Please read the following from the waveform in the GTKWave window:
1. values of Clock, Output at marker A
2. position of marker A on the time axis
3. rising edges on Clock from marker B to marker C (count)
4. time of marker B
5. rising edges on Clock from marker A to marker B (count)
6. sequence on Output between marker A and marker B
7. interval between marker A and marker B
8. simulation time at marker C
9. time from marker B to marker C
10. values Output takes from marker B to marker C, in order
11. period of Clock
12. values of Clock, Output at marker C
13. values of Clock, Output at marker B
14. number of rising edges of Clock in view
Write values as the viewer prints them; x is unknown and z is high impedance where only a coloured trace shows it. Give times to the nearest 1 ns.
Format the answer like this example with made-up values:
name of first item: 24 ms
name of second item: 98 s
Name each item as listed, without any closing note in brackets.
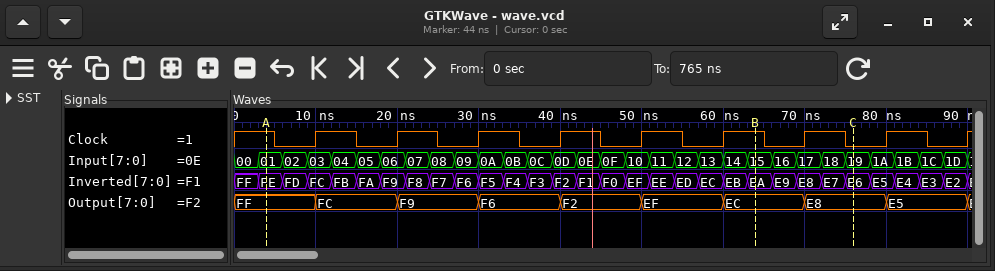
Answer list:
values of Clock, Output at marker A: Clock=1, Output=FF
position of marker A on the time axis: 4 ns
rising edges on Clock from marker B to marker C: 1
time of marker B: 64 ns
rising edges on Clock from marker A to marker B: 6
sequence on Output between marker A and marker B: FF, FC, F9, F6, F2, EF, EC
interval between marker A and marker B: 60 ns
simulation time at marker C: 76 ns
time from marker B to marker C: 12 ns
values Output takes from marker B to marker C, in order: EC, E8
period of Clock: 10 ns
values of Clock, Output at marker C: Clock=0, Output=E8
values of Clock, Output at marker B: Clock=1, Output=EC
number of rising edges of Clock in view: 9
